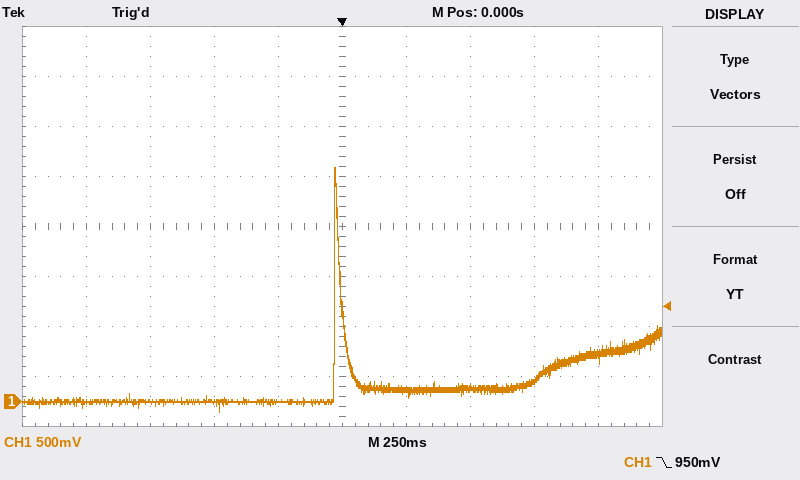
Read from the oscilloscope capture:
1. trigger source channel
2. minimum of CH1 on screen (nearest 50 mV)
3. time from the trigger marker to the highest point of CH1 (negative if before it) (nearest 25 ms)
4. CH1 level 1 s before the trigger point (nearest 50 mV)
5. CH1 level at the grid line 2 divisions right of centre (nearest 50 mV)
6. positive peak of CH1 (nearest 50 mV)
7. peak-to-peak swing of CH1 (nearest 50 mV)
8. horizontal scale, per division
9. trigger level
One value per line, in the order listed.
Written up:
CH1
-100 mV
-25 ms
0 mV
150 mV
2.35 V
2.45 V
250 ms
950 mV
